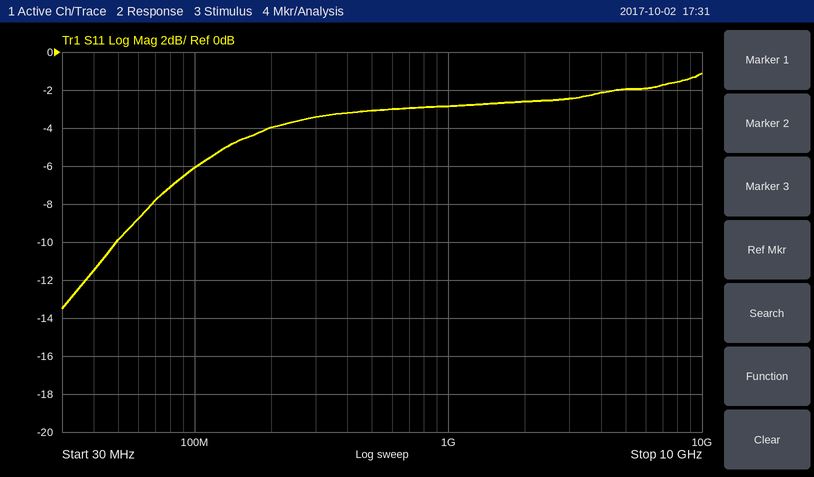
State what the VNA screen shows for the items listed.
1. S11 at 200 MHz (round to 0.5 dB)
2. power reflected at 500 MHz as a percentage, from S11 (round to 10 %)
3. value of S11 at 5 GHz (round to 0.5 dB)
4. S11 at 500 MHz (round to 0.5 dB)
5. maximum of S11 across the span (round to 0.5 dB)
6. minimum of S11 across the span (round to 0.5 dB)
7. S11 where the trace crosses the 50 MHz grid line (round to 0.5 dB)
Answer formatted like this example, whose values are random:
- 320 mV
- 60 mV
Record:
- -4.0 dB
- 50 %
- -2.0 dB
- -3.0 dB
- -1.0 dB
- -13.5 dB
- -10.0 dB
